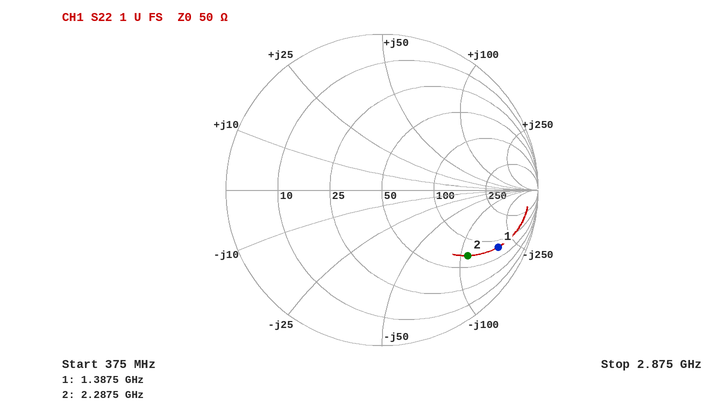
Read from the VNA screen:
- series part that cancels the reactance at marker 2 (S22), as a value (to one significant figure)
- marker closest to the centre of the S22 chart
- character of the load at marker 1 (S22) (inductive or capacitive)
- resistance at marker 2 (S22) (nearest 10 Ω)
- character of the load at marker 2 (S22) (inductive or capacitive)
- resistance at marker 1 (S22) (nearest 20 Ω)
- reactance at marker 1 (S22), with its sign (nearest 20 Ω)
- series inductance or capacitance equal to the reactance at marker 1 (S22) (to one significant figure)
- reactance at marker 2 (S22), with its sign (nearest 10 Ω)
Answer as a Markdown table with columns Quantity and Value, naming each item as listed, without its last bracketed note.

| Quantity | Value |
|---|---|
| series part that cancels the reactance at marker 2 (S22), as a value | 8 nH |
| marker closest to the centre of the S22 chart | marker 2 |
| character of the load at marker 1 (S22) | capacitive |
| resistance at marker 2 (S22) | 70 Ω |
| character of the load at marker 2 (S22) | capacitive |
| resistance at marker 1 (S22) | 80 Ω |
| reactance at marker 1 (S22), with its sign | -180 Ω |
| series inductance or capacitance equal to the reactance at marker 1 (S22) | 600 fF |
| reactance at marker 2 (S22), with its sign | -110 Ω |
